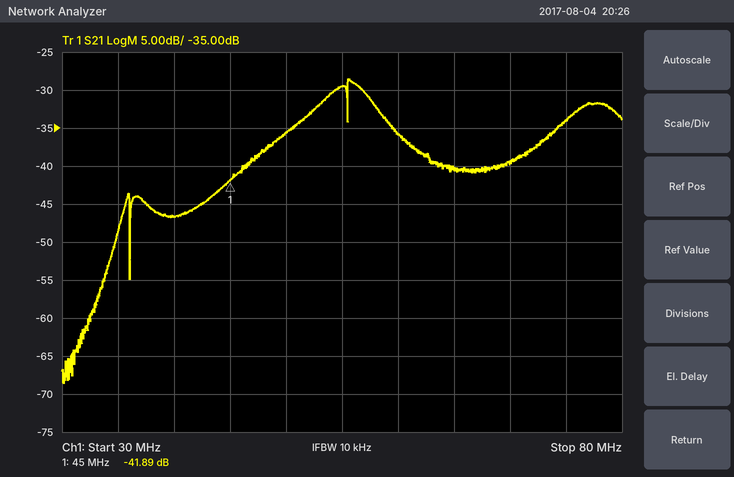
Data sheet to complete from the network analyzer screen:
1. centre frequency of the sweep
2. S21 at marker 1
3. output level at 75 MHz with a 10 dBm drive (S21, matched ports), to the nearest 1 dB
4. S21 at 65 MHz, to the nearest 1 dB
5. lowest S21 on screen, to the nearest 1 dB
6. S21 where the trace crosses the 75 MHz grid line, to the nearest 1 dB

55 MHz
-41.89 dB
-24 dBm
-40 dB
-69 dB
-34 dB
